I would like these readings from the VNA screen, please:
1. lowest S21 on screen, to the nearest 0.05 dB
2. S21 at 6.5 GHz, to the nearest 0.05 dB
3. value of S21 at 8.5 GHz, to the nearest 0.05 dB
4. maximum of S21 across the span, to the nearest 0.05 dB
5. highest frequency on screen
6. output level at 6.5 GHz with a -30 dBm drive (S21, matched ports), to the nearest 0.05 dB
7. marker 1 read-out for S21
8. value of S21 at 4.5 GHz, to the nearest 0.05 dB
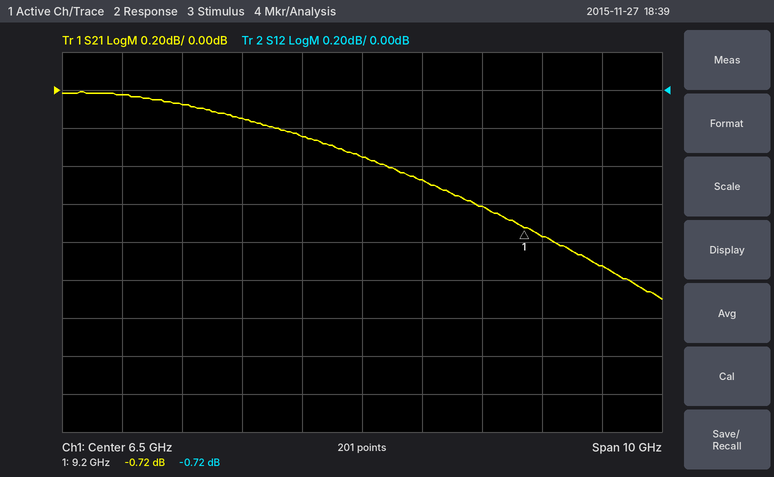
-1.10 dB
-0.35 dB
-0.60 dB
0.00 dB
11.5 GHz
-30.35 dBm
-0.72 dB
-0.15 dB
